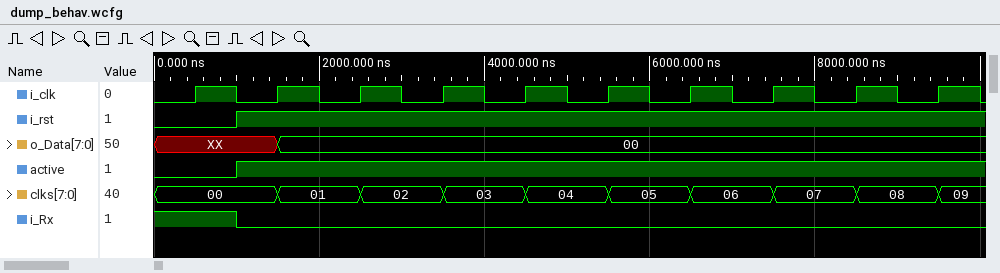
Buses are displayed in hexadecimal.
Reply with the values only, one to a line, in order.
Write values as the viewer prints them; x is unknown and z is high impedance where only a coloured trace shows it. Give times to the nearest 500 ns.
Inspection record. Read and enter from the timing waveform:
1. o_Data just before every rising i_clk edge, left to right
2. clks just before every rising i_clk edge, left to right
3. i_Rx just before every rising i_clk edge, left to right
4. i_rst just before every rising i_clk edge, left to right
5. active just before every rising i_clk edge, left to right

XX, XX, 00, 00, 00, 00, 00, 00, 00, 00
00, 00, 01, 02, 03, 04, 05, 06, 07, 08
1 0 0 0 0 0 0 0 0 0
0 1 1 1 1 1 1 1 1 1
0 1 1 1 1 1 1 1 1 1
